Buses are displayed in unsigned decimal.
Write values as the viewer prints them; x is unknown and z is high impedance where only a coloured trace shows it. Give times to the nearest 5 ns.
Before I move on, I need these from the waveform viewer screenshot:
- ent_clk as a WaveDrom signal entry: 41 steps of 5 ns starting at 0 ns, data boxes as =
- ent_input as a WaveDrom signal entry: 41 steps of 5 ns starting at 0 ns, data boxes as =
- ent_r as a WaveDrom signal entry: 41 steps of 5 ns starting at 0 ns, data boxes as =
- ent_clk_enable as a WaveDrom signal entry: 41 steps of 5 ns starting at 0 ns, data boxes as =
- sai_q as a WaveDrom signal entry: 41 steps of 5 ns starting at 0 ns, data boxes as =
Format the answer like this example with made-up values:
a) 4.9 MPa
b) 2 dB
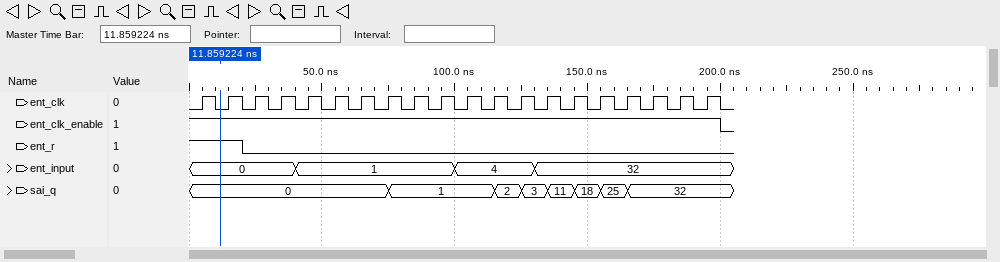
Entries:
a) {name: 'ent_clk', wave: '01010101010101010101010101010101010101010'}
b) {name: 'ent_input', wave: '=.......=...........=.....=..............', data: '0 1 4 32'}
c) {name: 'ent_r', wave: '1...0....................................'}
d) {name: 'ent_clk_enable', wave: '1.......................................0'}
e) {name: 'sai_q', wave: '=..............=.......=.=.=.=.=.=.......', data: '0 1 2 3 11 18 25 32'}
